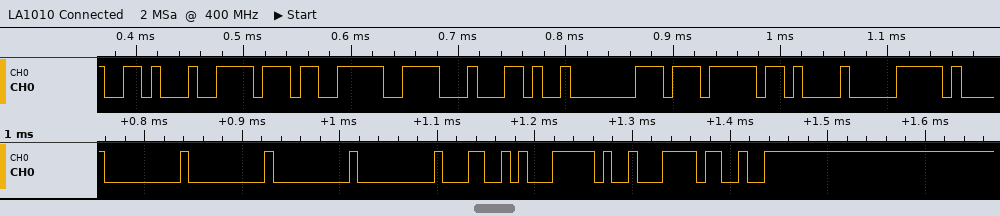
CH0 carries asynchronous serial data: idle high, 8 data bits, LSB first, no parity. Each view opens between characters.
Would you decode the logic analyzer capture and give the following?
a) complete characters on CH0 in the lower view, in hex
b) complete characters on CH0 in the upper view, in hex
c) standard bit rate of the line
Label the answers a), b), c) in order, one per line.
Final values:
a) 00, 00, 00, 00, 4C, 7C, E2, 93
b) 16, DE, F3, 1E, 2C, C0, F7, 0B, F0
c) 115200 baud
